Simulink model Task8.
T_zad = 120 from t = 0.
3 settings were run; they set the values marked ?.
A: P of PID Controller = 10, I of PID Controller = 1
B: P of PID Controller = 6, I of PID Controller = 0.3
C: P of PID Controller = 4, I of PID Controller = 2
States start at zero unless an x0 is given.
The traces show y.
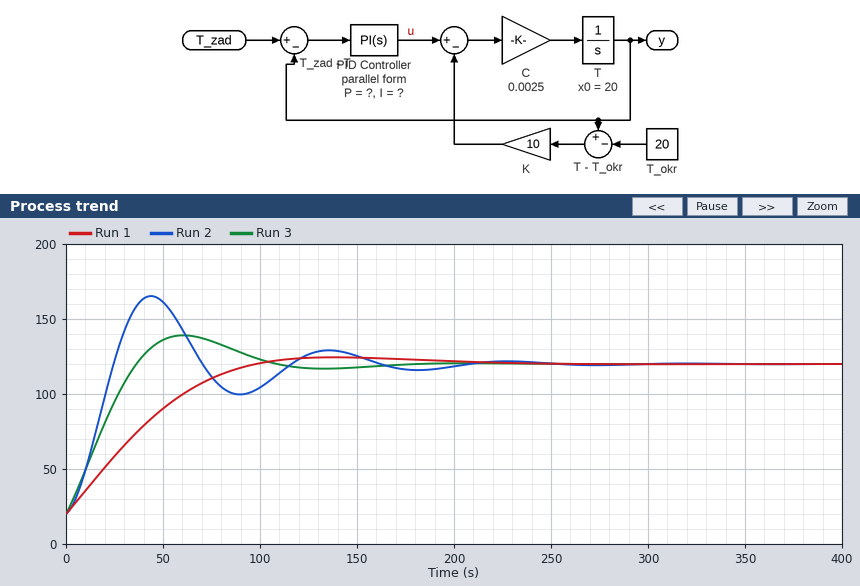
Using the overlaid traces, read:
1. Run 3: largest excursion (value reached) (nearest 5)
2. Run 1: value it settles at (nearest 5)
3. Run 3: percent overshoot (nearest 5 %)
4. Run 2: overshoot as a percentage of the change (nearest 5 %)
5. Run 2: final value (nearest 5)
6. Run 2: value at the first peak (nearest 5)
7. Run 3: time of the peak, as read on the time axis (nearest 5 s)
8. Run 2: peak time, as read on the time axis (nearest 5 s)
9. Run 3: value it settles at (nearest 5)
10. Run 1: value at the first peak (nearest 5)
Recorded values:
140
120
20 %
45 %
120
165
60 s
45 s
120
125
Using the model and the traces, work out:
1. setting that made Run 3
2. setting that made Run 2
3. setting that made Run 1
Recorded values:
A
C
B
